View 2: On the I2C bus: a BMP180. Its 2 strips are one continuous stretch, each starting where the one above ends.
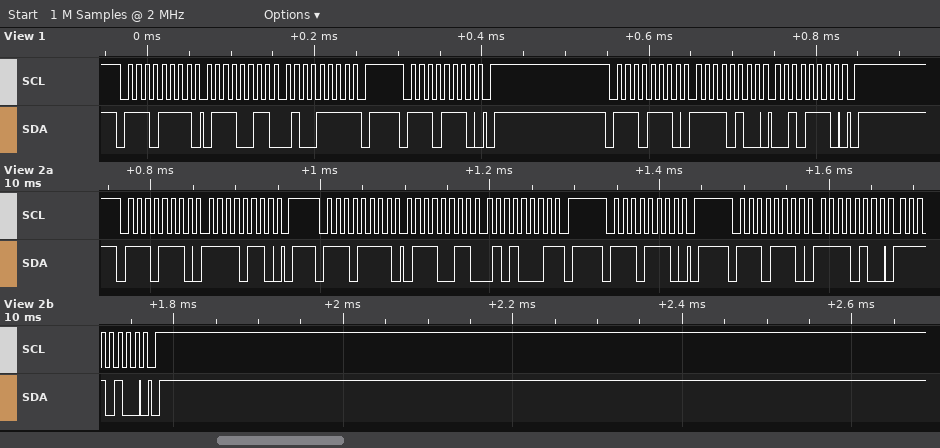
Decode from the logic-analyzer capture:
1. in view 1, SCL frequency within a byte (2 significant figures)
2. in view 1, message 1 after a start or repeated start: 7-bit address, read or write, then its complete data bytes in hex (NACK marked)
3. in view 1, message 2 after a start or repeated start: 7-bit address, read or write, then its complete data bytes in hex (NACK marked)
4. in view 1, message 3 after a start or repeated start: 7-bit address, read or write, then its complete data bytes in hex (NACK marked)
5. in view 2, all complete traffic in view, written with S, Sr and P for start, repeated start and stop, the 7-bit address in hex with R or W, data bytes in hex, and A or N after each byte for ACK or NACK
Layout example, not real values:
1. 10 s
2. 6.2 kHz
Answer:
1. 100 kHz
2. 0x77 read: 73 4F NACK
3. 0x77 write
4. 0x77 write: F4 2E
5. S 77W A F6 A P S 77R A 73 A 51 N P S 77W A P S 77W A F4 A F4 A P
